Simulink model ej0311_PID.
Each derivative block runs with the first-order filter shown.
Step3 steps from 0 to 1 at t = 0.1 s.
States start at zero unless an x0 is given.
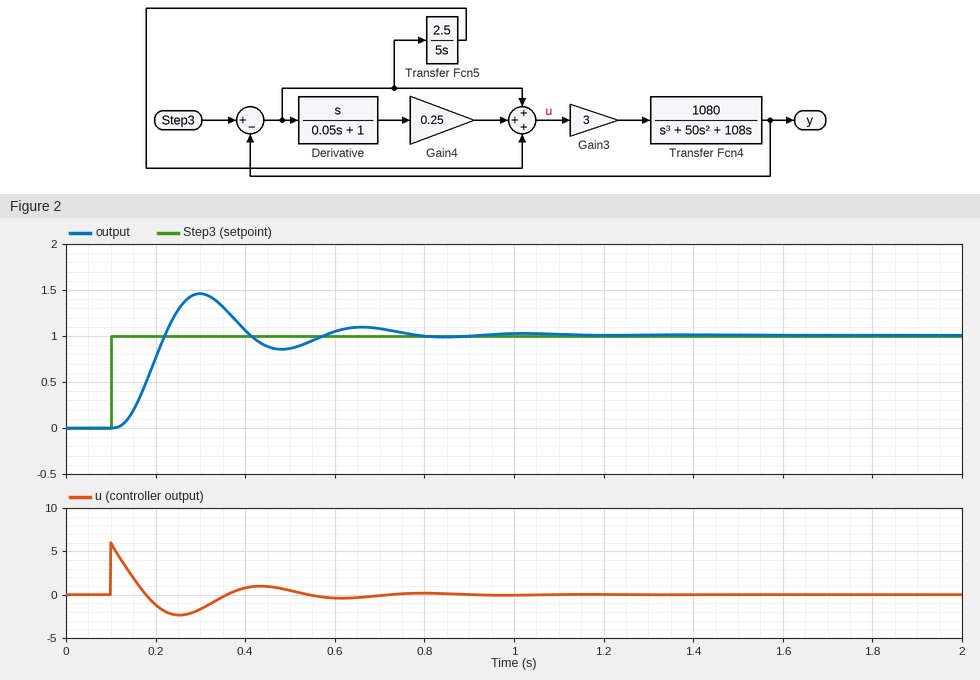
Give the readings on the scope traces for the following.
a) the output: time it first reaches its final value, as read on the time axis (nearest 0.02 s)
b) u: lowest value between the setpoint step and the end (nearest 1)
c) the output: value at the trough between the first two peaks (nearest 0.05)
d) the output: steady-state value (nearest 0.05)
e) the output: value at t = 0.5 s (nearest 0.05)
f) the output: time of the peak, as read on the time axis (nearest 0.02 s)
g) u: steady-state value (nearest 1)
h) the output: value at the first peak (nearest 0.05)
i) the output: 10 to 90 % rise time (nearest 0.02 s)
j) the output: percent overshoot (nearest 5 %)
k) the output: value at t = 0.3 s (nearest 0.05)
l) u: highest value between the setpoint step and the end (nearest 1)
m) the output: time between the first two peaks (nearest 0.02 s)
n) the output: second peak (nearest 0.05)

0.22 s
-2
0.85
1.00
0.85
0.30 s
0
1.45
0.08 s
45 %
1.45
6
0.36 s
1.10
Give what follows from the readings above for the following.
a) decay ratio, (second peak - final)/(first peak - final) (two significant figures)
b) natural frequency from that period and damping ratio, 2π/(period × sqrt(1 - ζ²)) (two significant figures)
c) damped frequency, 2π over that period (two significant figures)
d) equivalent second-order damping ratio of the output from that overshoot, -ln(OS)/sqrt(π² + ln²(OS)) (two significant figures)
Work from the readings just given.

0.22
18 rad/s
17 rad/s
0.25
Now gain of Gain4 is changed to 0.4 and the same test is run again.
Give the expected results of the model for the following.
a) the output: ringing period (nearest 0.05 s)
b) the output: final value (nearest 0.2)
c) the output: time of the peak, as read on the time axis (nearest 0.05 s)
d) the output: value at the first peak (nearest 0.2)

0.30 s
1.0
0.25 s
1.6
